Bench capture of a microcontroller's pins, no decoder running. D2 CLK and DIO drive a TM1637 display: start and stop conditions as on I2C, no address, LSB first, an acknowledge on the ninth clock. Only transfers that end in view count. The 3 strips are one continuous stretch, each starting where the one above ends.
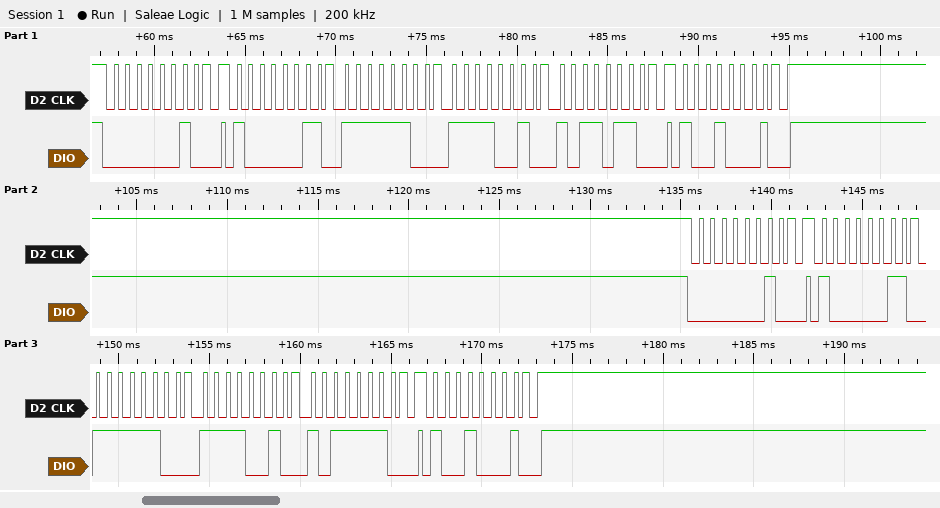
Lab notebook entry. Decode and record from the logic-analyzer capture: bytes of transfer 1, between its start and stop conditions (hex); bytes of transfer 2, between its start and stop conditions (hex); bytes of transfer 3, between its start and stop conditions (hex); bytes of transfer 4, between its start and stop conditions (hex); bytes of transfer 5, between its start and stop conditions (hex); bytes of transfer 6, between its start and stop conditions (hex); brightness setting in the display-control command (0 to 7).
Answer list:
40
C1 3F 4F 6D
89
40
C1 3F 4F 7D
89
1
